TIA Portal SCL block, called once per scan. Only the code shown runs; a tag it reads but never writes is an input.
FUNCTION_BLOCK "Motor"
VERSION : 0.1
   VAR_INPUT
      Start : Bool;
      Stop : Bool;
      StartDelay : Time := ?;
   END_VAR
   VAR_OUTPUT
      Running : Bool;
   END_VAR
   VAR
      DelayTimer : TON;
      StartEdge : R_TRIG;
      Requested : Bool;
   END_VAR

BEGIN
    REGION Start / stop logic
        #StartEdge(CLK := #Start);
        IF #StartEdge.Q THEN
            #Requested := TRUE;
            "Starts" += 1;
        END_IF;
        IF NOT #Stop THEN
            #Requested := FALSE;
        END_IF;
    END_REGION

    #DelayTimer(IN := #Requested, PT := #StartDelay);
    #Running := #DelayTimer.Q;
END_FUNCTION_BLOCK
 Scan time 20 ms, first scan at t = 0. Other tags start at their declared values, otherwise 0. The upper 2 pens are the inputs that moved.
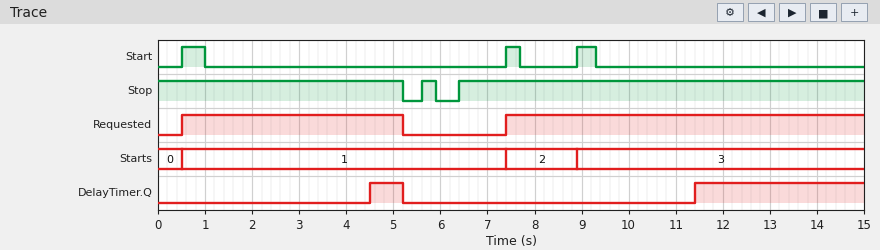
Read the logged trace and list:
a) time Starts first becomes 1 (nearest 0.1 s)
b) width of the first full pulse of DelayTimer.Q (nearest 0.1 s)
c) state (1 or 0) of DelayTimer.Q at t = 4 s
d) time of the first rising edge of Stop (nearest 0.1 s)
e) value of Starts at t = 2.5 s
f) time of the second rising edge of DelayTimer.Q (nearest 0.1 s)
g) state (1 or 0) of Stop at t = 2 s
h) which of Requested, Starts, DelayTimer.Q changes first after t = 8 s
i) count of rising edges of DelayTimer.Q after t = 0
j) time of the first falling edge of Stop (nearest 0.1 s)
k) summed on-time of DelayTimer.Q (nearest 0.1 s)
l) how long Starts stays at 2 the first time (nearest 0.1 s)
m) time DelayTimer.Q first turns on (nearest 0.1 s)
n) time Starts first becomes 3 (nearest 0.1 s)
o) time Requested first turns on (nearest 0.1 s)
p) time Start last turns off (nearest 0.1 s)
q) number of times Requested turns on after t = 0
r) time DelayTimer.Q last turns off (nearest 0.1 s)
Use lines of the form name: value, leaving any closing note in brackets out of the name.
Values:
time Starts first becomes 1: 0.5 s
width of the first full pulse of DelayTimer.Q: 0.7 s
state (1 or 0) of DelayTimer.Q at t = 4 s: 0
time of the first rising edge of Stop: 5.6 s
value of Starts at t = 2.5 s: 1
time of the second rising edge of DelayTimer.Q: 11.4 s
state (1 or 0) of Stop at t = 2 s: 1
which of Requested, Starts, DelayTimer.Q changes first after t = 8 s: Starts
count of rising edges of DelayTimer.Q after t = 0: 2
time of the first falling edge of Stop: 5.2 s
summed on-time of DelayTimer.Q: 4.3 s
how long Starts stays at 2 the first time: 1.5 s
time DelayTimer.Q first turns on: 4.5 s
time Starts first becomes 3: 8.9 s
time Requested first turns on: 0.5 s
time Start last turns off: 9.3 s
number of times Requested turns on after t = 0: 2
time DelayTimer.Q last turns off: 5.2 s
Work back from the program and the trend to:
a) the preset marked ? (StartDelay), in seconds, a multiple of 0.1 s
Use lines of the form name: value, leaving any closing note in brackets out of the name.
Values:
the preset marked ? (StartDelay), in seconds, a multiple of 0.1 s: 4.0 s
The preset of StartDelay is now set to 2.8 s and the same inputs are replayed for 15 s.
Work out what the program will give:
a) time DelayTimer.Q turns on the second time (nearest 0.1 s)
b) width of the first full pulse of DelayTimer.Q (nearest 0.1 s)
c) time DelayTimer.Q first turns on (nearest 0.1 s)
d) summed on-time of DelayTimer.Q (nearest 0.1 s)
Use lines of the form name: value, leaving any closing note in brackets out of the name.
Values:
time DelayTimer.Q turns on the second time: 10.2 s
width of the first full pulse of DelayTimer.Q: 1.9 s
time DelayTimer.Q first turns on: 3.3 s
summed on-time of DelayTimer.Q: 6.7 s
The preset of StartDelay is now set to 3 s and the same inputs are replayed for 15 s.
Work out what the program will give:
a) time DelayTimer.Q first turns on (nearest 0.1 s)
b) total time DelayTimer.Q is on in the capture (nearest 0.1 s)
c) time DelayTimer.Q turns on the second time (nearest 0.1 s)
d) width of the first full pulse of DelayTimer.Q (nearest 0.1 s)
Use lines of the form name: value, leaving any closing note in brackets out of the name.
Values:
time DelayTimer.Q first turns on: 3.5 s
total time DelayTimer.Q is on in the capture: 6.3 s
time DelayTimer.Q turns on the second time: 10.4 s
width of the first full pulse of DelayTimer.Q: 1.7 s
